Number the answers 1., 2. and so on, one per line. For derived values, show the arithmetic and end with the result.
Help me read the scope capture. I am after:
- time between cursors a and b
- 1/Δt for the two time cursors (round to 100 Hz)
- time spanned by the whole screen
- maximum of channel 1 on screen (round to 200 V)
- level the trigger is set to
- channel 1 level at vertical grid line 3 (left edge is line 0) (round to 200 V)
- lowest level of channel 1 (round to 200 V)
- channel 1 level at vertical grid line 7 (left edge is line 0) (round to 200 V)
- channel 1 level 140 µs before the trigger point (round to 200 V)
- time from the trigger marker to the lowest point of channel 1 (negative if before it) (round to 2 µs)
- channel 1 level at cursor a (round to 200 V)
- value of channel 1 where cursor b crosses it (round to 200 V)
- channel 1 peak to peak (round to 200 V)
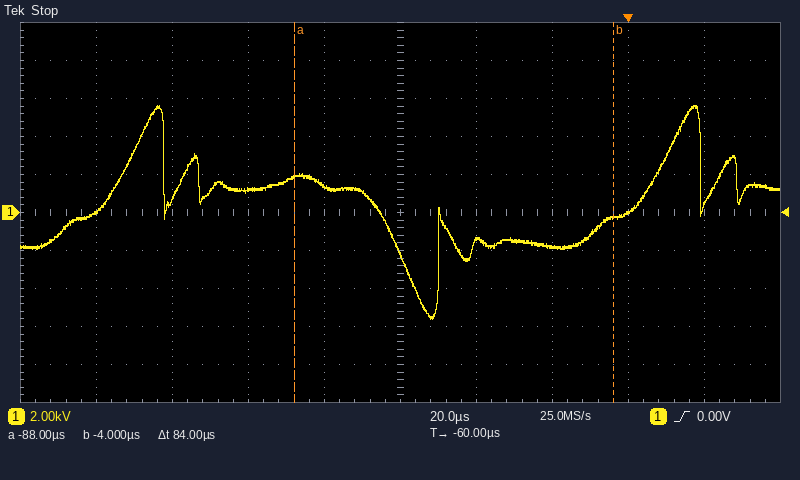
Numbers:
1. 84 µs
2. 1 / 84 µs ≈ 11.9 kHz
3. 200 µs
4. 5.6 kV
5. 0.00 V
6. 1.2 kV
7. -5.6 kV
8. -1.8 kV
9. 0.0 kV
10. -52 µs
11. 1.8 kV
12. -200 V
13. 5.6 kV − (-5.6 kV) = 11.2 kV
